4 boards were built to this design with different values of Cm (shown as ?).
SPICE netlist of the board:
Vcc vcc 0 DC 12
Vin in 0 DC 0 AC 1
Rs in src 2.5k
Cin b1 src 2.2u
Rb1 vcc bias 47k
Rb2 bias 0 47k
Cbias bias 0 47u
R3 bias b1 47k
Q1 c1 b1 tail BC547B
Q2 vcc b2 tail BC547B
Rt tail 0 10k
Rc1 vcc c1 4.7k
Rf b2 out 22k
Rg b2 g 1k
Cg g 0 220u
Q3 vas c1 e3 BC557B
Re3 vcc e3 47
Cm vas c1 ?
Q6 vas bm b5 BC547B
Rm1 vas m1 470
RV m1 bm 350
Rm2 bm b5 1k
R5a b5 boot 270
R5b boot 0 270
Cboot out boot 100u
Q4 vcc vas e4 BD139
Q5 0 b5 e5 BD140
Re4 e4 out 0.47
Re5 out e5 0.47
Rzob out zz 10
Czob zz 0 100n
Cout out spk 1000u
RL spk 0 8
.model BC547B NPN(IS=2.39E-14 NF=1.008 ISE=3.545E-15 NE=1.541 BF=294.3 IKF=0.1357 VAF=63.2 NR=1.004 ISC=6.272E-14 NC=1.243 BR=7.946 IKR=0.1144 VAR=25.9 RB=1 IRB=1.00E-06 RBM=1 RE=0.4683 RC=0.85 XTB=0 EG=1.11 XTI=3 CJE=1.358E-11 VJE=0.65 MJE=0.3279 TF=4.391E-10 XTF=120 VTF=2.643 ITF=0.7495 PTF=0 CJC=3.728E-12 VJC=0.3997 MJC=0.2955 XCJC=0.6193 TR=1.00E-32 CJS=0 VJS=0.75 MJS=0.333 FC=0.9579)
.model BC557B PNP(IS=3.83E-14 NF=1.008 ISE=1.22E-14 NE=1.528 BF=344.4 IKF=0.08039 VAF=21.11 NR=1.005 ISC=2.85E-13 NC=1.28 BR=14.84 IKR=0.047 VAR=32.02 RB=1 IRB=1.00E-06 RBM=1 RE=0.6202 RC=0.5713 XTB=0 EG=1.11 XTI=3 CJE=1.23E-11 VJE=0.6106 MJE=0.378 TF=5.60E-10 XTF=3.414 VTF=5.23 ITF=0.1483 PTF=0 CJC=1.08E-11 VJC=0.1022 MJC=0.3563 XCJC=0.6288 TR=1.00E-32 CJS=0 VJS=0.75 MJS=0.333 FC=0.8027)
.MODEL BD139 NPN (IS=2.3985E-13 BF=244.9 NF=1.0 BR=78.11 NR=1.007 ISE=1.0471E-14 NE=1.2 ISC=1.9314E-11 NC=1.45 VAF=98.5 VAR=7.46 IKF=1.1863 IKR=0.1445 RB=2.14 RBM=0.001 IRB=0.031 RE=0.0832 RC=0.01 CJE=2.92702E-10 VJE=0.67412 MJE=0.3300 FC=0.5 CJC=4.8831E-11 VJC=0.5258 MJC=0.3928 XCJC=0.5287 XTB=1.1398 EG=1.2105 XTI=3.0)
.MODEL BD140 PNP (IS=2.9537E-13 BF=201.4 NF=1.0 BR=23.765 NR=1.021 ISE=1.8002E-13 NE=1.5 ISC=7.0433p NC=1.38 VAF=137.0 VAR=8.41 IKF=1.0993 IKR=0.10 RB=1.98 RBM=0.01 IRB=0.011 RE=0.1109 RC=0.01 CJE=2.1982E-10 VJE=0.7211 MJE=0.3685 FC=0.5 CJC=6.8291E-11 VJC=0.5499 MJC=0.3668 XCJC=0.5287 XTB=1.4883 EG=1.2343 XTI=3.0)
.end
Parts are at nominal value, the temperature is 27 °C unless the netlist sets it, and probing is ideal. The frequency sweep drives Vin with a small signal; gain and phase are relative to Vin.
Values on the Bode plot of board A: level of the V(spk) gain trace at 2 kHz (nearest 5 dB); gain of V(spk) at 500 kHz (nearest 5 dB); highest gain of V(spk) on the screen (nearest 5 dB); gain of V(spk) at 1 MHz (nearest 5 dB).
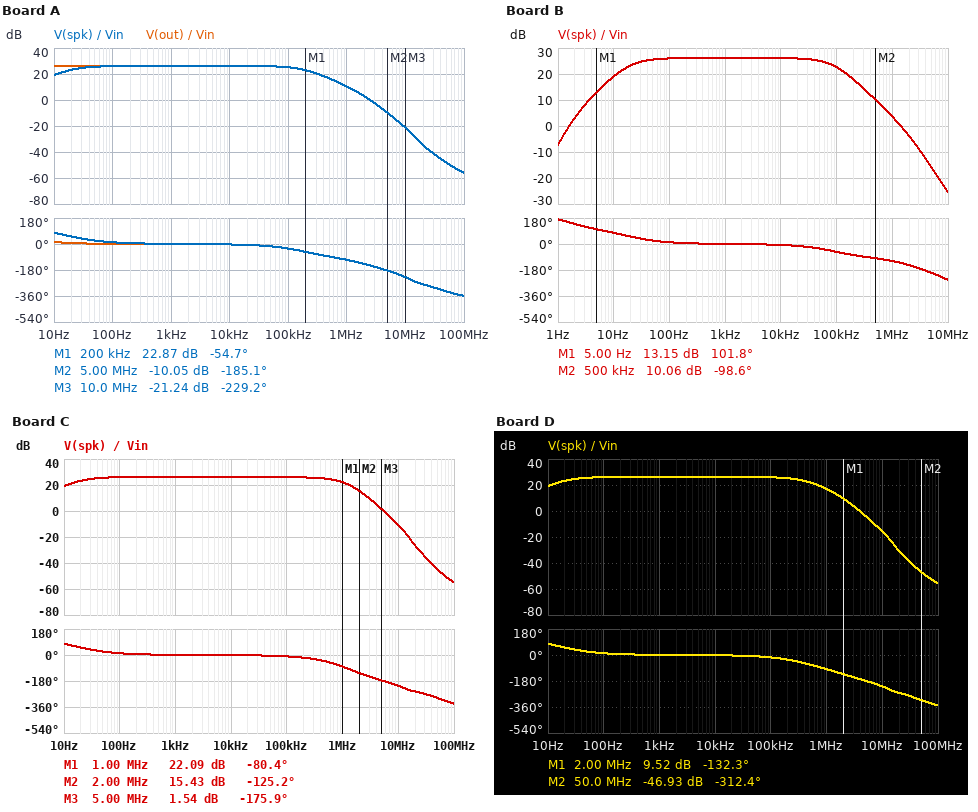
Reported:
25 dB
15 dB
25 dB
10 dB
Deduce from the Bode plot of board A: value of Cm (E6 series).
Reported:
150 pF
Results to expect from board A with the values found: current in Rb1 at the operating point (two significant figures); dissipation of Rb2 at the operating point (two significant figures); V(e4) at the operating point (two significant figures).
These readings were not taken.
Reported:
130 µA
760 µW
6.0 V
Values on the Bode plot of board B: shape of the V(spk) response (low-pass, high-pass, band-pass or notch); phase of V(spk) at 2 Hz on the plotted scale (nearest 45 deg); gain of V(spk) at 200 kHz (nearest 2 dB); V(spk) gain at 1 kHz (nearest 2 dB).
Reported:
band-pass
135 deg
18 dB
26 dB
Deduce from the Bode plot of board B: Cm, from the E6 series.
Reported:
330 pF
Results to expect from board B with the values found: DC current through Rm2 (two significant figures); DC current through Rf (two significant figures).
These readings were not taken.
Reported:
700 µA
840 nA
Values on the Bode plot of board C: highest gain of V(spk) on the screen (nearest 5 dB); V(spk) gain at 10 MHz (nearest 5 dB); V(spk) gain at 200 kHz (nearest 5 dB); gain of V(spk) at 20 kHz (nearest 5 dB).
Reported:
25 dB
-10 dB
25 dB
25 dB
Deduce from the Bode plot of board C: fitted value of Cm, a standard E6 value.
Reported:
33 pF
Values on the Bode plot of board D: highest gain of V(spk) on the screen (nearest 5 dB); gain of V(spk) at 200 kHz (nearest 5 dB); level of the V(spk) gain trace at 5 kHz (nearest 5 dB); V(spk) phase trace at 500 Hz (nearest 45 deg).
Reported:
25 dB
25 dB
25 dB
0 deg
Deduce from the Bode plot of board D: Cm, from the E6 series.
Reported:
68 pF
